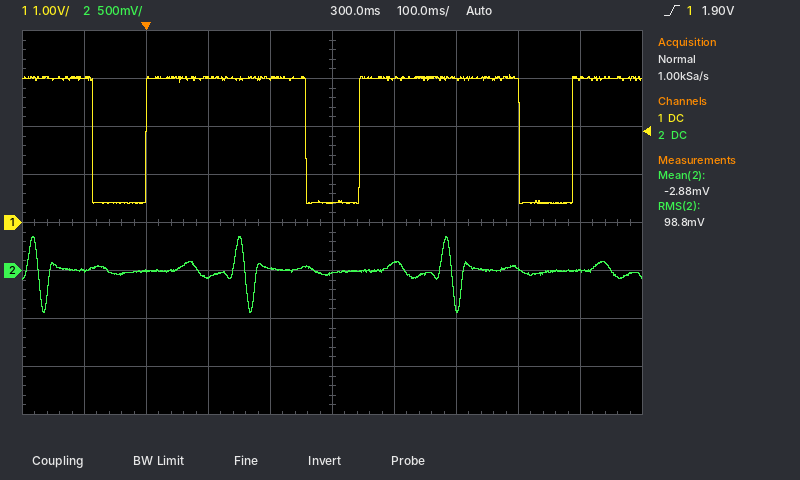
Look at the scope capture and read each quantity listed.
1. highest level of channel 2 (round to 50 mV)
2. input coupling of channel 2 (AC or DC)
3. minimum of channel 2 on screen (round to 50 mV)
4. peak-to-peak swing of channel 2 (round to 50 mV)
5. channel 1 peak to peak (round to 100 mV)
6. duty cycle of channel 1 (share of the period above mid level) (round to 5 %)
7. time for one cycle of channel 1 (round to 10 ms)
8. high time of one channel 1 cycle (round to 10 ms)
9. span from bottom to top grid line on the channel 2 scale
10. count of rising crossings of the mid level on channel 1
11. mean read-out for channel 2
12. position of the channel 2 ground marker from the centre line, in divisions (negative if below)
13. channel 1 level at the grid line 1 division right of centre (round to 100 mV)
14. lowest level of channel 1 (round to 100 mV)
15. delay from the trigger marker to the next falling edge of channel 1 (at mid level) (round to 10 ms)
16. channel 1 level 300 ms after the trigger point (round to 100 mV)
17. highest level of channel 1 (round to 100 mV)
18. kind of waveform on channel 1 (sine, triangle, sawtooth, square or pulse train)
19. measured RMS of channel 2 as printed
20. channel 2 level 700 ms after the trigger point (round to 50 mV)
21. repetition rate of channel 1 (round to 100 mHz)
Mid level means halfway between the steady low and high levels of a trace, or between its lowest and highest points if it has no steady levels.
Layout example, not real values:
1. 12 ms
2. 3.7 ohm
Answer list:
1. 350 mV
2. DC
3. -450 mV
4. 800 mV
5. 2.7 V
6. 75 %
7. 340 ms
8. 260 ms
9. 4 V
10. 3
11. -2.88 mV
12. -1.0 div
13. 3.0 V
14. 400 mV
15. 260 ms
16. 400 mV
17. 3.1 V
18. pulse train
19. 98.8 mV
20. 0 mV
21. 2.9 Hz
